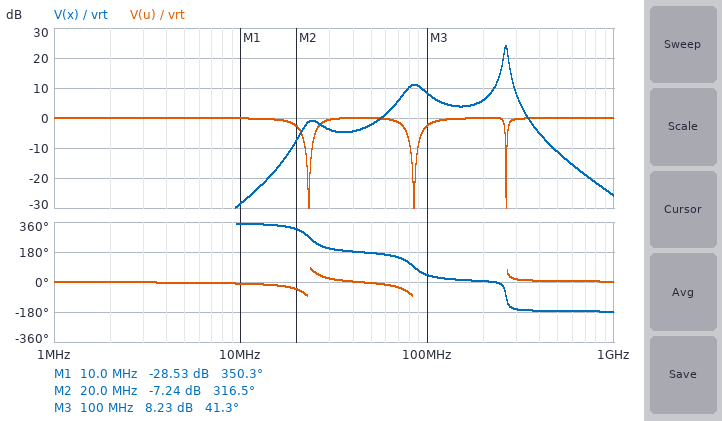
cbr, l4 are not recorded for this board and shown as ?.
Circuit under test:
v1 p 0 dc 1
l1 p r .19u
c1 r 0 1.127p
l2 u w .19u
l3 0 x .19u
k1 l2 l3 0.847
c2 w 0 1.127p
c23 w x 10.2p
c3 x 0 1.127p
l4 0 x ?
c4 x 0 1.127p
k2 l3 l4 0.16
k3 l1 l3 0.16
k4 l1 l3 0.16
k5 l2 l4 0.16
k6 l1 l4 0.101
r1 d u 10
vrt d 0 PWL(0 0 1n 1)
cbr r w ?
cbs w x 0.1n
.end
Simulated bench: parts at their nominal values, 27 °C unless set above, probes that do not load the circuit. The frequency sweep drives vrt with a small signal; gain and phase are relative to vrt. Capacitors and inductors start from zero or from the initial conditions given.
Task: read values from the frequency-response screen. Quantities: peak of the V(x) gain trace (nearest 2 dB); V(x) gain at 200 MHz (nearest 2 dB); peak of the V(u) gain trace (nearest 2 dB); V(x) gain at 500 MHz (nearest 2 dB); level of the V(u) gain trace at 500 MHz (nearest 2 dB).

24 dB
6 dB
0 dB
-12 dB
0 dB
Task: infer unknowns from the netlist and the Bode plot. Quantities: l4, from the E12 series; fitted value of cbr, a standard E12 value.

470 nH
120 pF
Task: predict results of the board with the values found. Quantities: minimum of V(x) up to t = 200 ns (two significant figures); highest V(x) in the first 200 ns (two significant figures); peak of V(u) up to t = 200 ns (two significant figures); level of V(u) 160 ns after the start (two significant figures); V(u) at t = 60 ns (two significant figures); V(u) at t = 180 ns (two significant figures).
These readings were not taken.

-1.5 V
1.7 V
1.2 V
1.0 V
980 mV
1.0 V
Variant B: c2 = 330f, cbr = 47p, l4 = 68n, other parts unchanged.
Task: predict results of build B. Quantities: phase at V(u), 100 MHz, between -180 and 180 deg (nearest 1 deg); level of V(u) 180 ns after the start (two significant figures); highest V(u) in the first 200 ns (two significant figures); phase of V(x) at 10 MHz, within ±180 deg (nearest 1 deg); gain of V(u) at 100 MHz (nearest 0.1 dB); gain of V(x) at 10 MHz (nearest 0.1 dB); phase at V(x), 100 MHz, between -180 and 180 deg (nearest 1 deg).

-55 deg
1.0 V
1.1 V
-6 deg
-4.8 dB
-51.0 dB
125 deg
